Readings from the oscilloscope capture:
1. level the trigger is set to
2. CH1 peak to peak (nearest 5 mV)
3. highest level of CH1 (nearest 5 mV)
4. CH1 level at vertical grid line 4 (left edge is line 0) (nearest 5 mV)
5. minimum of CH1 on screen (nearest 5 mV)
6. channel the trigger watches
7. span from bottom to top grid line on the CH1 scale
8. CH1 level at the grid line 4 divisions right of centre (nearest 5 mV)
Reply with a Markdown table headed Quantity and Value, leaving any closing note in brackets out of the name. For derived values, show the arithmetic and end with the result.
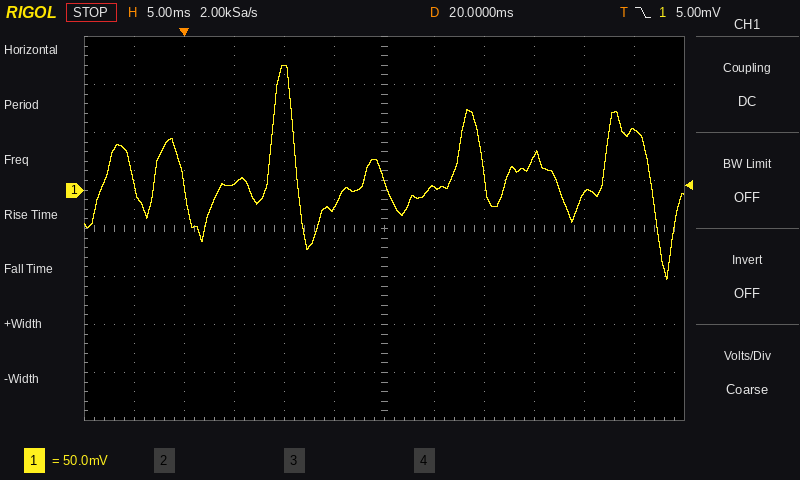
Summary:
| Quantity | Value |
|---|---|
| level the trigger is set to | 5.00 mV |
| CH1 peak to peak | 130 mV − (-95 mV) = 225 mV |
| highest level of CH1 | 130 mV |
| CH1 level at vertical grid line 4 (left edge is line 0) | 130 mV |
| minimum of CH1 on screen | -95 mV |
| channel the trigger watches | CH1 |
| span from bottom to top grid line on the CH1 scale | 400 mV |
| CH1 level at the grid line 4 divisions right of centre | -5 mV |
